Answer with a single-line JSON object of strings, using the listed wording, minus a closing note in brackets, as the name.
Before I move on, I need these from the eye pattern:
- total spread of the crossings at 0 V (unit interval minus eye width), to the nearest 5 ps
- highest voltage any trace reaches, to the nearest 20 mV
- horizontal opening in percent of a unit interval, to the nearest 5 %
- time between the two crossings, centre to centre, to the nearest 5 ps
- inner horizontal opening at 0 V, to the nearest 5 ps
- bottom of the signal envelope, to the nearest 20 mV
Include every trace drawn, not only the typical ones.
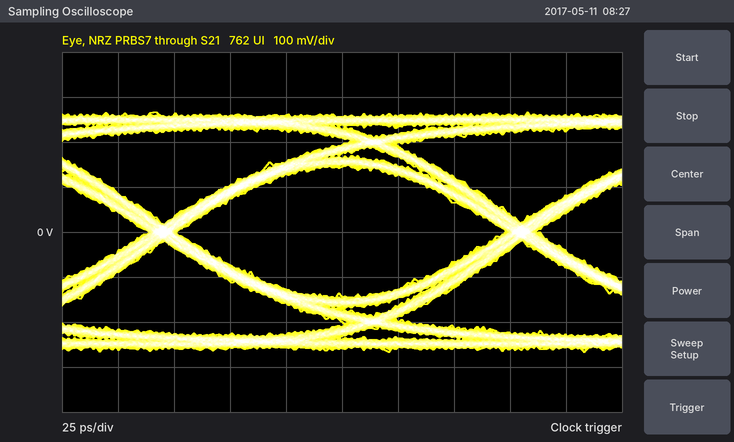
{"total spread of the crossings at 0 V (unit interval minus eye width), to the nearest 5 ps": "15 ps", "highest voltage any trace reaches, to the nearest 20 mV": "260 mV", "horizontal opening in percent of a unit interval, to the nearest 5 %": "90 %", "time between the two crossings, centre to centre, to the nearest 5 ps": "160 ps", "inner horizontal opening at 0 V, to the nearest 5 ps": "145 ps", "bottom of the signal envelope, to the nearest 20 mV": "-260 mV"}
